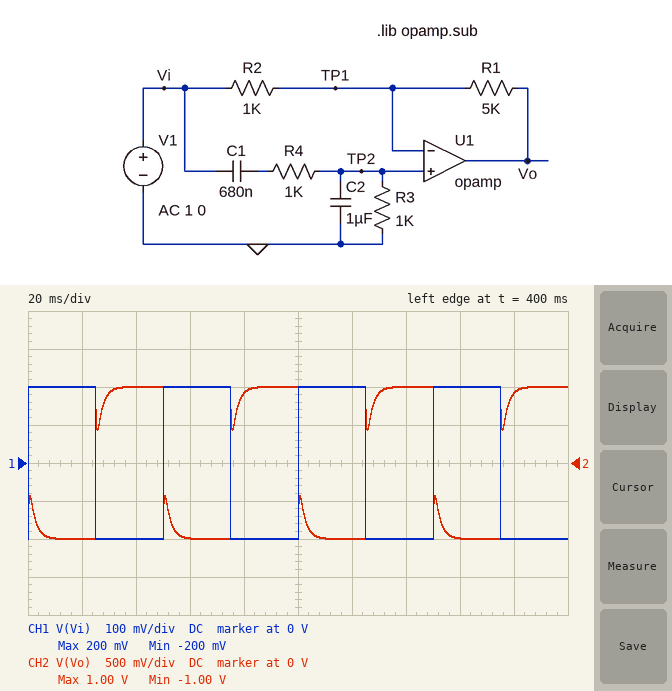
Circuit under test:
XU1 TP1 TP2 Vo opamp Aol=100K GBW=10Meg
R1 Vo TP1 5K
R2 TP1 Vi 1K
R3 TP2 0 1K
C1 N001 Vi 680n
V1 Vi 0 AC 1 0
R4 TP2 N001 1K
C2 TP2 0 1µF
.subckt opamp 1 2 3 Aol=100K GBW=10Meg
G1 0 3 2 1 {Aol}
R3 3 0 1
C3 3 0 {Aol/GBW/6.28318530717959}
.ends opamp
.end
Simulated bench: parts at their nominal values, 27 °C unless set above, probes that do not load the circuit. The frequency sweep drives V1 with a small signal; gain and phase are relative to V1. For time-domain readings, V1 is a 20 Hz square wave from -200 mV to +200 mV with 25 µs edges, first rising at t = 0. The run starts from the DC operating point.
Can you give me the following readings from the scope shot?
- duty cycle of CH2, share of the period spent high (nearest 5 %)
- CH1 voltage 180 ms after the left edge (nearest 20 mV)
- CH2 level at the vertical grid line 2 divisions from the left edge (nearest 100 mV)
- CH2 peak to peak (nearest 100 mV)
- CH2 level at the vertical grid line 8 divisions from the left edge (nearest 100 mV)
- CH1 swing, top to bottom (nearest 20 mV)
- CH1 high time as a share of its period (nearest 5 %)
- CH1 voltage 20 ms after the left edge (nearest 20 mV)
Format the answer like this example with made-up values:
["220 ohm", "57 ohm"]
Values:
["50 %", "-200 mV", "1.0 V", "2.0 V", "-1.0 V", "400 mV", "50 %", "200 mV"]
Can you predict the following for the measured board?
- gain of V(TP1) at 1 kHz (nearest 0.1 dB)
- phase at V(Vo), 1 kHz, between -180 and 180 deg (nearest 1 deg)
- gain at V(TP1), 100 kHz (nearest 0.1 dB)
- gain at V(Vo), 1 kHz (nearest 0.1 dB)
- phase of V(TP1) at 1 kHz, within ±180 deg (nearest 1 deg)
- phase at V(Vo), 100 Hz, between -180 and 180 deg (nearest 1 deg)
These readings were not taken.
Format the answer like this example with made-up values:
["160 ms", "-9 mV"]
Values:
["-16.9 dB", "-171 deg", "-26.3 dB", "13.3 dB", "-60 deg", "169 deg"]
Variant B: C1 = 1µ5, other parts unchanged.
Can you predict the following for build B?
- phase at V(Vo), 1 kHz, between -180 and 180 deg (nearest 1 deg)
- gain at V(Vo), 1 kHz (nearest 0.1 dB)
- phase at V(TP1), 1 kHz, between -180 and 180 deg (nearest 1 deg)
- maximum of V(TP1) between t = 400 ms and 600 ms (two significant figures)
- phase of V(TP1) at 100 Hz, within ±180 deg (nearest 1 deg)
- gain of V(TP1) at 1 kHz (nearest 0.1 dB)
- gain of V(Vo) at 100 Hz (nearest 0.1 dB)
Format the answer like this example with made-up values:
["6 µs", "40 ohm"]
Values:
["-170 deg", "13.5 dB", "-67 deg", "130 mV", "9 deg", "-16.6 dB", "9.0 dB"]
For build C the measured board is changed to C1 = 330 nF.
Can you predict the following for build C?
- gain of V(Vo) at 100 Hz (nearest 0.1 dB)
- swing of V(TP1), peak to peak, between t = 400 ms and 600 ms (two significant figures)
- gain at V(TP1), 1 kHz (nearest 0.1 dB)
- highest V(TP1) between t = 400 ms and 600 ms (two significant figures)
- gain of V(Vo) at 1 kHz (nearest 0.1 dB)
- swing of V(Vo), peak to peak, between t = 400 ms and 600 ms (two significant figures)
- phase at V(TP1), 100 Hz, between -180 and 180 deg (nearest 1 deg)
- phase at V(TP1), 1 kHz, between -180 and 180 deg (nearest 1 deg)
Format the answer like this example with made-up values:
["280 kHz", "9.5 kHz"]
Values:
["12.7 dB", "130 mV", "-17.7 dB", "65 mV", "13.1 dB", "2.0 V", "40 deg", "-49 deg"]
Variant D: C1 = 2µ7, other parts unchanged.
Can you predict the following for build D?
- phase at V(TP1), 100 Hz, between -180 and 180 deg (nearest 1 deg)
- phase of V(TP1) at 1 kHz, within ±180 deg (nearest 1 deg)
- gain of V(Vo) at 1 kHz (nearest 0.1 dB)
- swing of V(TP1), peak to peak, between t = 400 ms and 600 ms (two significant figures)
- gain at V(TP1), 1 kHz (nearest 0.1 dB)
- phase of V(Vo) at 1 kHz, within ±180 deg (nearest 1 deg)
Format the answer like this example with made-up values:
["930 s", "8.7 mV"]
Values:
["-1 deg", "-69 deg", "13.5 dB", "290 mV", "-16.5 dB", "-170 deg"]
